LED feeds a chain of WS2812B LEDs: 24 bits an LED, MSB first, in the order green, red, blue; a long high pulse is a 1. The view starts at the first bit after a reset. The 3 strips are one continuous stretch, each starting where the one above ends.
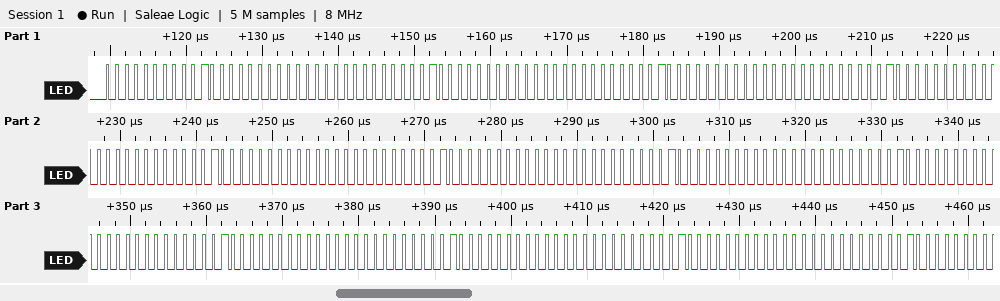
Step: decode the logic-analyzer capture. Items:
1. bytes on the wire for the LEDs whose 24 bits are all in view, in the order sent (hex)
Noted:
00 20 00 00 20 00 00 20 00 00 20 00 00 20 00 00 20 00 00 20 00 00 20 00 00 20 00 00 20 00 00 20 00
